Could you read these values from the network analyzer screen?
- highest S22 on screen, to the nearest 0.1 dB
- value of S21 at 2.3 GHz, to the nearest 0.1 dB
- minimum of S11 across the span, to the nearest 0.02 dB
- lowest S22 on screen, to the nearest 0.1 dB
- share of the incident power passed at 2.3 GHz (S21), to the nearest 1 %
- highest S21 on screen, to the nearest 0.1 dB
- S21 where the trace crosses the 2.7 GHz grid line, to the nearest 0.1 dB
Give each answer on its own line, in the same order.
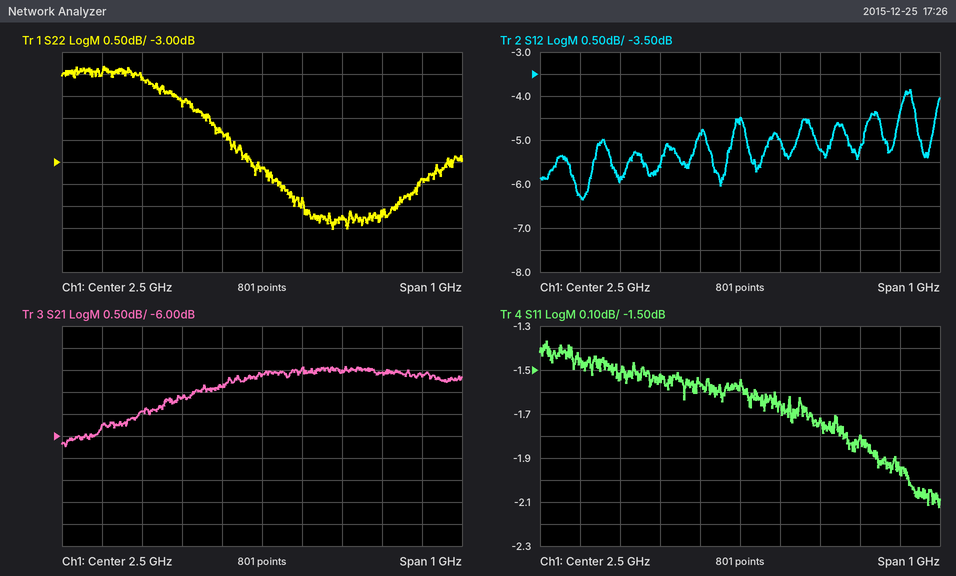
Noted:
-0.8 dB
-5.1 dB
-2.12 dB
-4.5 dB
31 %
-4.4 dB
-4.5 dB
